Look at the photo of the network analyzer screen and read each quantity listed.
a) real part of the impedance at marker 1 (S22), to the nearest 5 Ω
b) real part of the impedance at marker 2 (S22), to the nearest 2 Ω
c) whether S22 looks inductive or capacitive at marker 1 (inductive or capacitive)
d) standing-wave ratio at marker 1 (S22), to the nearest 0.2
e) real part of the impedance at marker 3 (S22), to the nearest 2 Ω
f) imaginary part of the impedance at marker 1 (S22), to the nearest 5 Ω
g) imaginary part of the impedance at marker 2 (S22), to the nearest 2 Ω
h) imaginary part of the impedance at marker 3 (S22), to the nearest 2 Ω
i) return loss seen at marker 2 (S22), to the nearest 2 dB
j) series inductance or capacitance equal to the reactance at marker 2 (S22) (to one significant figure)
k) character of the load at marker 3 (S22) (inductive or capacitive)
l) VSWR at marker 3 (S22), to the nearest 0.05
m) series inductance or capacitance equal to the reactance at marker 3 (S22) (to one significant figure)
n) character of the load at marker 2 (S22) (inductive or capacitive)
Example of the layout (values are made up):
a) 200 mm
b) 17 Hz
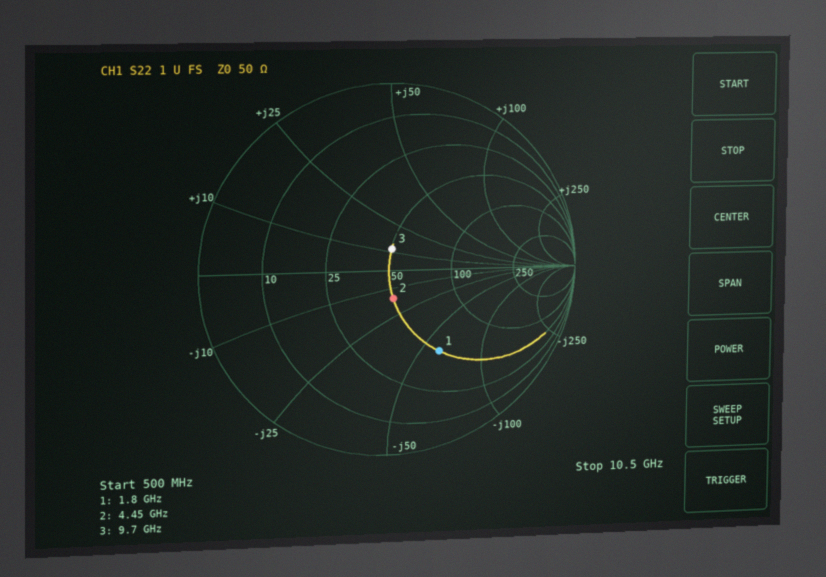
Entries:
a) 50 Ω
b) 50 Ω
c) capacitive
d) 3.2
e) 50 Ω
f) -60 Ω
g) -16 Ω
h) +12 Ω
i) 16 dB
j) 2 pF
k) inductive
l) 1.25
m) 200 pH
n) capacitive
